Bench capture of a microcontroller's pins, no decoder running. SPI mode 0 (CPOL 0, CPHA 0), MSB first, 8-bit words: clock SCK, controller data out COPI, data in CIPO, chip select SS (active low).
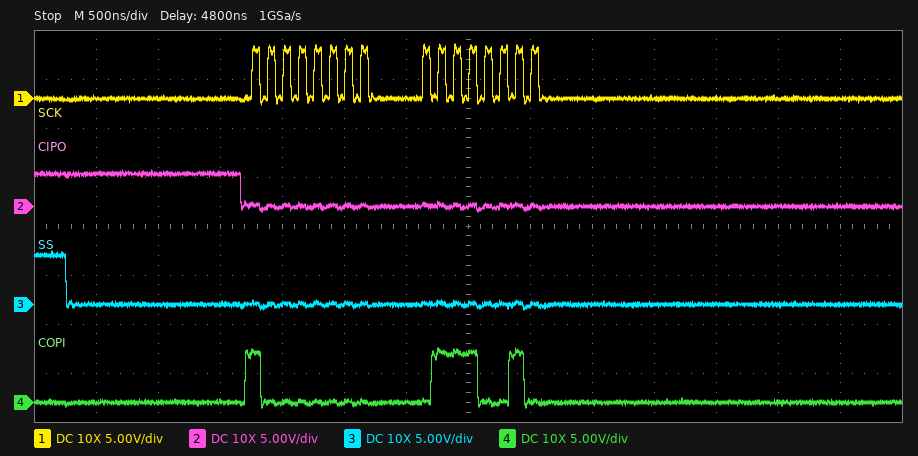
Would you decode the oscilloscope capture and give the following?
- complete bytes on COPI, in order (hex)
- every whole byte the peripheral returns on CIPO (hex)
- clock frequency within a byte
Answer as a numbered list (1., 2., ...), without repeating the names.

1. 80 72
2. 00 00
3. 8 MHz
